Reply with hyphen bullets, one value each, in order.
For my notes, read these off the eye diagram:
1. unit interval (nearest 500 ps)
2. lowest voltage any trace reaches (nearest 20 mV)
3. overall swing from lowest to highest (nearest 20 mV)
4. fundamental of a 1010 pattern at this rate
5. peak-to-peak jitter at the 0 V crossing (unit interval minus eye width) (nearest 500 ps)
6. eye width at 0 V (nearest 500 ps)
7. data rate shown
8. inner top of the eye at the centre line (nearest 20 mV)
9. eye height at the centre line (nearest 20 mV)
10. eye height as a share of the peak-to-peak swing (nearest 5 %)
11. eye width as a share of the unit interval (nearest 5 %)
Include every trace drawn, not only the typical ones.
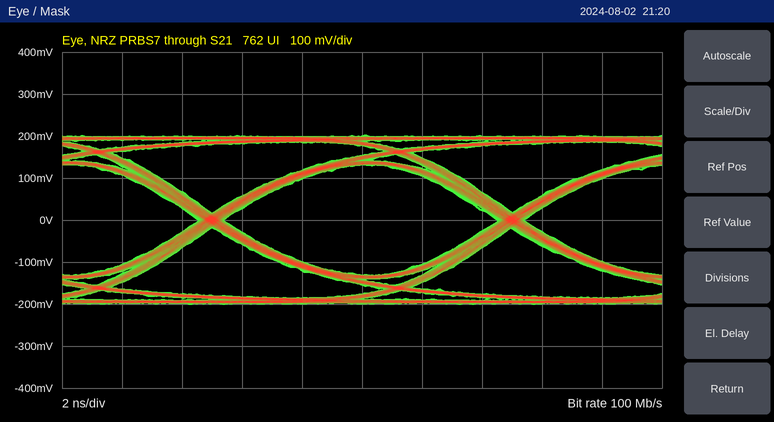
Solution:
- 10.0 ns
- -200 mV
- 400 mV
- 50 MHz
- 1.0 ns
- 9.0 ns
- 100 Mb/s
- 140 mV
- 260 mV
- 65 %
- 90 %
